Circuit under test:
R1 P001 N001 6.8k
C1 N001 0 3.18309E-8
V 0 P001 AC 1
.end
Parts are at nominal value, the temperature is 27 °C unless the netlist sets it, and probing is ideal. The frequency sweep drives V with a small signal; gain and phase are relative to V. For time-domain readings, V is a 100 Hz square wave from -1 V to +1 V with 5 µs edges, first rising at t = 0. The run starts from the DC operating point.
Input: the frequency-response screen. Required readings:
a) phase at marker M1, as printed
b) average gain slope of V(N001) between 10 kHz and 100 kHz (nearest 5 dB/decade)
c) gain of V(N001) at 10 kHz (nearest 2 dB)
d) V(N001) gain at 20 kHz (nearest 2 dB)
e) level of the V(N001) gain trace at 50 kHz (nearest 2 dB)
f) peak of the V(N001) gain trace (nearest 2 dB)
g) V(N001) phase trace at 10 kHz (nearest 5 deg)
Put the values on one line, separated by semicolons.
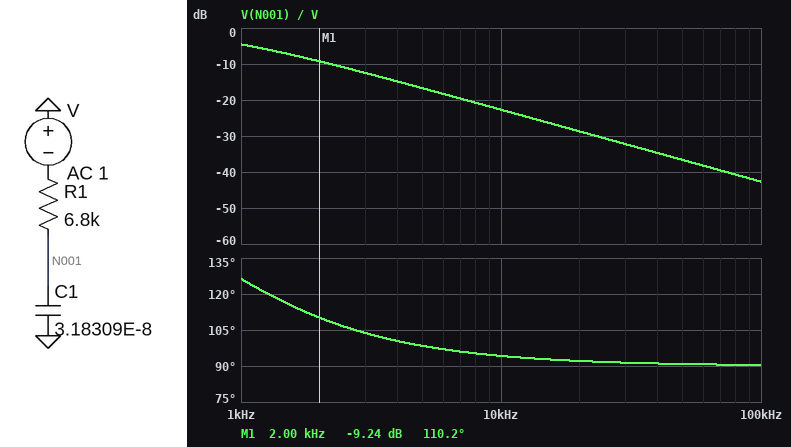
110.2 deg; -20 dB/decade; -22 dB; -28 dB; -36 dB; -4 dB; 95 deg
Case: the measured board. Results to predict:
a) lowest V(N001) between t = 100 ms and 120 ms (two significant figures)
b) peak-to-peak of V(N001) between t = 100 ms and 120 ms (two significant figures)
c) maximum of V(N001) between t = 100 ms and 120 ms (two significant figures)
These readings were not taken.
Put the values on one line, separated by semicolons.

-1.0 V; 2.0 V; 1.0 V
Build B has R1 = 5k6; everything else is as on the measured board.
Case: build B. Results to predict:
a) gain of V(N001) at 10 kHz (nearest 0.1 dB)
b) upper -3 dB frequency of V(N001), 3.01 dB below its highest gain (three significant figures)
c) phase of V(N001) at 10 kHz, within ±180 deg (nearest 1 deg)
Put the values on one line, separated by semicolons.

-21.0 dB; 893 Hz; 95 deg
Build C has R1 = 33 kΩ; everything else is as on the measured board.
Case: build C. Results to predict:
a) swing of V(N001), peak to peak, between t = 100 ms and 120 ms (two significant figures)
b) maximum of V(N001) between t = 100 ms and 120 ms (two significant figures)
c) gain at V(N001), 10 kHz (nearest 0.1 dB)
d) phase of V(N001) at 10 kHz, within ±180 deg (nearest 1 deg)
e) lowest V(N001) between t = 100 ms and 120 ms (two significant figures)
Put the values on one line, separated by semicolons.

2.0 V; 980 mV; -36.4 dB; 91 deg; -980 mV
